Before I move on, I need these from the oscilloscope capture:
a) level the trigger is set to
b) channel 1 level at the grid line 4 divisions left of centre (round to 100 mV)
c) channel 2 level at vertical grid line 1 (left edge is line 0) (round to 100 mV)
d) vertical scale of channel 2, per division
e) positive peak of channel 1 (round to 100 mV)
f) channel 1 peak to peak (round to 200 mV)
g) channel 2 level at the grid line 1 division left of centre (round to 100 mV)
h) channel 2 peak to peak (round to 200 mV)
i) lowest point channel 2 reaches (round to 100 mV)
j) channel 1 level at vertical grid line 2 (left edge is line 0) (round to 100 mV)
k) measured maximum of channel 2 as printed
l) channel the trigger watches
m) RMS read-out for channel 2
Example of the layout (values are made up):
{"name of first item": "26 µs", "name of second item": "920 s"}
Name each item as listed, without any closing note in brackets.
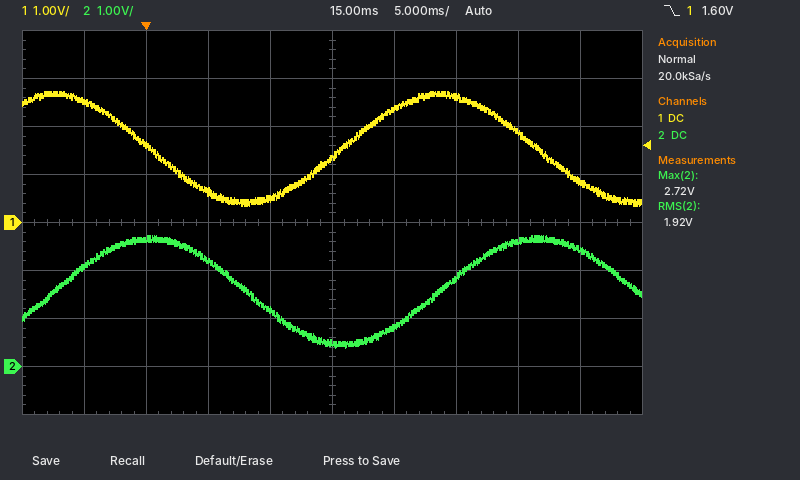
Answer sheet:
{"level the trigger is set to": "1.60 V", "channel 1 level at the grid line 4 divisions left of centre": "2.5 V", "channel 2 level at vertical grid line 1 (left edge is line 0)": "2.1 V", "vertical scale of channel 2, per division": "1 V", "positive peak of channel 1": "2.7 V", "channel 1 peak to peak": "2.4 V", "channel 2 level at the grid line 1 division left of centre": "1.2 V", "channel 2 peak to peak": "2.4 V", "lowest point channel 2 reaches": "400 mV", "channel 1 level at vertical grid line 2 (left edge is line 0)": "1.6 V", "measured maximum of channel 2 as printed": "2.72 V", "channel the trigger watches": "channel 1", "RMS read-out for channel 2": "1.92 V"}
